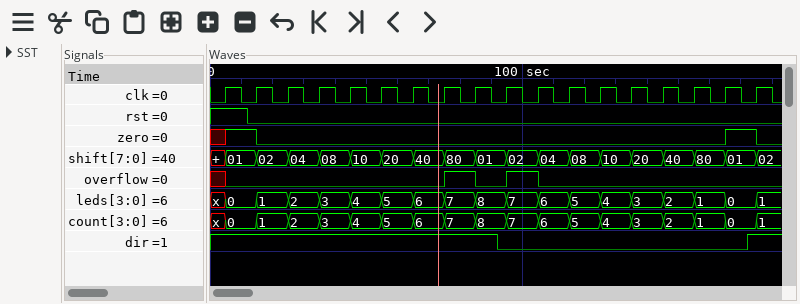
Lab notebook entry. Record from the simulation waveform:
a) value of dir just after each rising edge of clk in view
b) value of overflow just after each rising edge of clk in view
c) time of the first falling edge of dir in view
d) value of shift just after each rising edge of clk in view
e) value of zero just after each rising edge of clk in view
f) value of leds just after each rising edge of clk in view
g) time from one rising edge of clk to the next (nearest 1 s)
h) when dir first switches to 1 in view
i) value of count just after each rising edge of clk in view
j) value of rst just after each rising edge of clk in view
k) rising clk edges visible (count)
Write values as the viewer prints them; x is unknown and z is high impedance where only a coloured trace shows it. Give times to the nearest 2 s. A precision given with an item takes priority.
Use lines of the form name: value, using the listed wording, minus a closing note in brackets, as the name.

value of dir just after each rising edge of clk in view: 1 1 1 1 1 1 1 1 1 0 0 0 0 0 0 0 0 1
value of overflow just after each rising edge of clk in view: 0 0 0 0 0 0 0 1 0 1 0 0 0 0 0 0 0 0
time of the first falling edge of dir in view: 92 s
value of shift just after each rising edge of clk in view: 01, 02, 04, 08, 10, 20, 40, 80, 01, 02, 04, 08, 10, 20, 40, 80, 01, 02
value of zero just after each rising edge of clk in view: 1 0 0 0 0 0 0 0 0 0 0 0 0 0 0 0 1 0
value of leds just after each rising edge of clk in view: 0, 1, 2, 3, 4, 5, 6, 7, 8, 7, 6, 5, 4, 3, 2, 1, 0, 1
time from one rising edge of clk to the next: 10 s
when dir first switches to 1 in view: 172 s
value of count just after each rising edge of clk in view: 0, 1, 2, 3, 4, 5, 6, 7, 8, 7, 6, 5, 4, 3, 2, 1, 0, 1
value of rst just after each rising edge of clk in view: 1 0 0 0 0 0 0 0 0 0 0 0 0 0 0 0 0 0
rising clk edges visible: 18
